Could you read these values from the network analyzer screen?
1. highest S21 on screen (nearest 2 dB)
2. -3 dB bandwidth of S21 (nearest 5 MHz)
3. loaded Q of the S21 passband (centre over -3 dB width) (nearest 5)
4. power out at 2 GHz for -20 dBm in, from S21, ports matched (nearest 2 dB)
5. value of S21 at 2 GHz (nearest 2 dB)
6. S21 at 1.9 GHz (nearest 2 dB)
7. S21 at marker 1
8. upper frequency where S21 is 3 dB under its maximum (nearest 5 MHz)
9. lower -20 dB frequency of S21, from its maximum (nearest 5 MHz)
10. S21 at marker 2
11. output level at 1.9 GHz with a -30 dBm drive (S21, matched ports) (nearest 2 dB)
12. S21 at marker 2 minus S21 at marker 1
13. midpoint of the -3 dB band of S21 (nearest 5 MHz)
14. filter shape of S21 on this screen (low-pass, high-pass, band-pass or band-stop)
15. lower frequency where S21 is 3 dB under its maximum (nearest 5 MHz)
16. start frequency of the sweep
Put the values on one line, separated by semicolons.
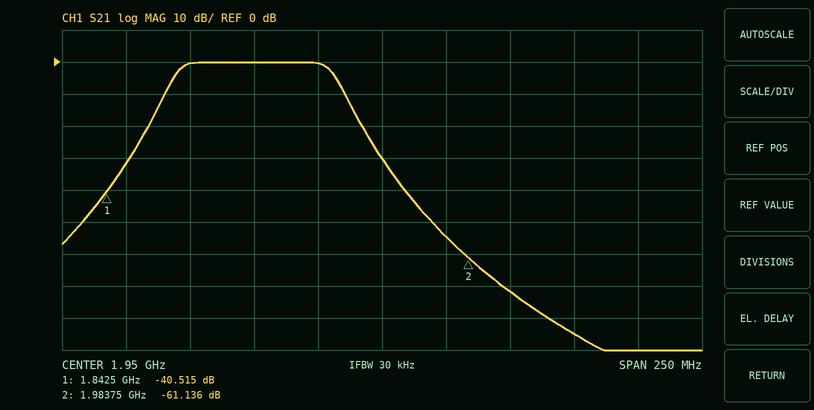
0 dB; 60 MHz; 30; -92 dBm; -72 dB; 0 dB; -40.515 dB; 1.930 GHz; 1.860 GHz; -61.136 dB; -30 dBm; -20.621 dB; 1.900 GHz; band-pass; 1.870 GHz; 1.825 GHz
